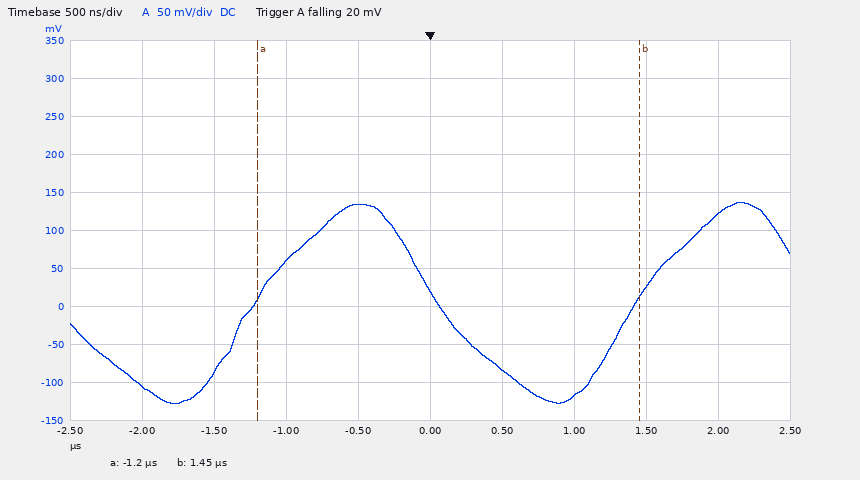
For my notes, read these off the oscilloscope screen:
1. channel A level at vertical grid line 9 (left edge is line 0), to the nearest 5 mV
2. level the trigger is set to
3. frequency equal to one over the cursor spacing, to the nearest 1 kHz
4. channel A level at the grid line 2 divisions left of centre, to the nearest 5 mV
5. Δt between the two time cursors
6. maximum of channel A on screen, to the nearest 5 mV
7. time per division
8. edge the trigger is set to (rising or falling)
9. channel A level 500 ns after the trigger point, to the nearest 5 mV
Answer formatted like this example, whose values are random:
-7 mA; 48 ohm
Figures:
120 mV; 20 mV; 377 kHz; 60 mV; 2.65 µs; 135 mV; 500 ns; falling; -85 mV
